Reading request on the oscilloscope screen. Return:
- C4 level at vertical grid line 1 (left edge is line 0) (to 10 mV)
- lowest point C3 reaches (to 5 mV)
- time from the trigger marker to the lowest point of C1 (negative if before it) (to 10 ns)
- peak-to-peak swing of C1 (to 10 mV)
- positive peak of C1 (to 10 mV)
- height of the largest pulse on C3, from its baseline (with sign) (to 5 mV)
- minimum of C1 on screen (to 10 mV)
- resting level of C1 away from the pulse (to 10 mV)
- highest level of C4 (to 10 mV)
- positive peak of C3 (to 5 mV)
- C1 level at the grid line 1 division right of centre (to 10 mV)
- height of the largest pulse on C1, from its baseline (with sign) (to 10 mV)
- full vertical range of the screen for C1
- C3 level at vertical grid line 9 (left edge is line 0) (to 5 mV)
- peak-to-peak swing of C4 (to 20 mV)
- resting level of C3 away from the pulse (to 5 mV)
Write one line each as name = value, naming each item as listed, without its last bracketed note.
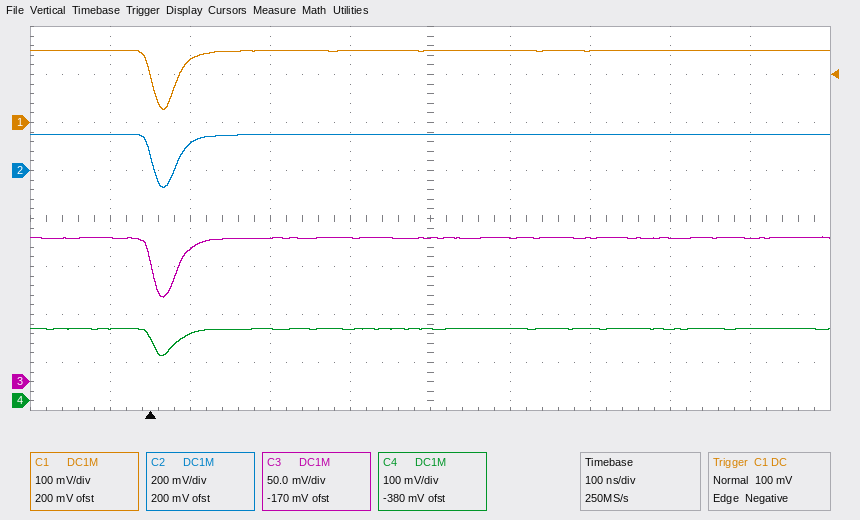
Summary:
C4 level at vertical grid line 1 (left edge is line 0) = 150 mV
lowest point C3 reaches = 90 mV
time from the trigger marker to the lowest point of C1 (negative if before it) = +20 ns
peak-to-peak swing of C1 = 120 mV
positive peak of C1 = 150 mV
height of the largest pulse on C3, from its baseline (with sign) = -60 mV
minimum of C1 on screen = 30 mV
resting level of C1 away from the pulse = 150 mV
highest level of C4 = 150 mV
positive peak of C3 = 150 mV
C1 level at the grid line 1 division right of centre = 150 mV
height of the largest pulse on C1, from its baseline (with sign) = -120 mV
full vertical range of the screen for C1 = 800 mV
C3 level at vertical grid line 9 (left edge is line 0) = 150 mV
peak-to-peak swing of C4 = 60 mV
resting level of C3 away from the pulse = 150 mV
